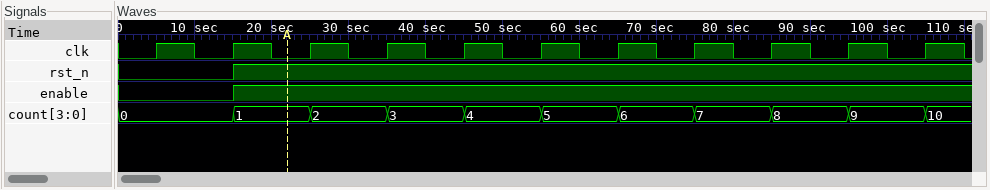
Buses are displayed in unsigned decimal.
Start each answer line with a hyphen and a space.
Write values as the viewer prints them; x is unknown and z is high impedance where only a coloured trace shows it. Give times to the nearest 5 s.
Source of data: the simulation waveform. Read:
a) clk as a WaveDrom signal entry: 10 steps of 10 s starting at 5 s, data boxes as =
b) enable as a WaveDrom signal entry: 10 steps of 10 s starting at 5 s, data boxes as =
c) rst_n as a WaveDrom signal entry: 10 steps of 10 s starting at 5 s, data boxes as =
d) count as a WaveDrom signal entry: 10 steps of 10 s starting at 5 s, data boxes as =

- {name: 'clk', wave: 'p.........'}
- {name: 'enable', wave: '01........'}
- {name: 'rst_n', wave: '01........'}
- {name: 'count', wave: '==========', data: '0 1 2 3 4 5 6 7 8 9'}
